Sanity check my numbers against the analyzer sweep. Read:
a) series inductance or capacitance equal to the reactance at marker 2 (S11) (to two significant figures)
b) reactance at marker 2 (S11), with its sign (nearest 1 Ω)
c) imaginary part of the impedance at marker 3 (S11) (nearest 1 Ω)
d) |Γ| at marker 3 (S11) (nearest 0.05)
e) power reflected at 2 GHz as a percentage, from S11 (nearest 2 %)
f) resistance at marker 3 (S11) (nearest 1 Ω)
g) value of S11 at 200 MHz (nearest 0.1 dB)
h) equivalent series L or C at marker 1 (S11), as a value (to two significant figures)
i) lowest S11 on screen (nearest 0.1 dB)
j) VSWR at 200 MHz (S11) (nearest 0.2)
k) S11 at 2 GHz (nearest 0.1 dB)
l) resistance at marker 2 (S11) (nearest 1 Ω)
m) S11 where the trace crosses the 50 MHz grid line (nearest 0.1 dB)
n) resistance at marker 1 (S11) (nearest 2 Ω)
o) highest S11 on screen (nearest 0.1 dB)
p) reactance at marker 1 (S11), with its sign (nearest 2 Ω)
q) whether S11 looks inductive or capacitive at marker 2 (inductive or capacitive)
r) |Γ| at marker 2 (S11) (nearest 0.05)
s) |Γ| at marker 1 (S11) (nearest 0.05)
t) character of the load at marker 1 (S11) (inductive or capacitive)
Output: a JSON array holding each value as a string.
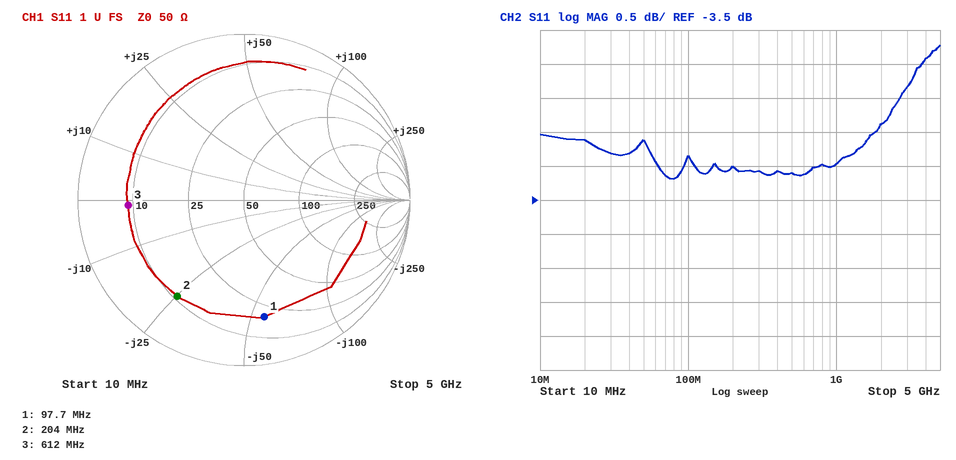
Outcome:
["31 pF", "-25 Ω", "-1 Ω", "0.70", "58 %", "9 Ω", "-3.0 dB", "29 pF", "-3.2 dB", "5.8", "-2.4 dB", "11 Ω", "-2.6 dB", "20 Ω", "-1.2 dB", "-56 Ω", "capacitive", "0.70", "0.70", "capacitive"]
